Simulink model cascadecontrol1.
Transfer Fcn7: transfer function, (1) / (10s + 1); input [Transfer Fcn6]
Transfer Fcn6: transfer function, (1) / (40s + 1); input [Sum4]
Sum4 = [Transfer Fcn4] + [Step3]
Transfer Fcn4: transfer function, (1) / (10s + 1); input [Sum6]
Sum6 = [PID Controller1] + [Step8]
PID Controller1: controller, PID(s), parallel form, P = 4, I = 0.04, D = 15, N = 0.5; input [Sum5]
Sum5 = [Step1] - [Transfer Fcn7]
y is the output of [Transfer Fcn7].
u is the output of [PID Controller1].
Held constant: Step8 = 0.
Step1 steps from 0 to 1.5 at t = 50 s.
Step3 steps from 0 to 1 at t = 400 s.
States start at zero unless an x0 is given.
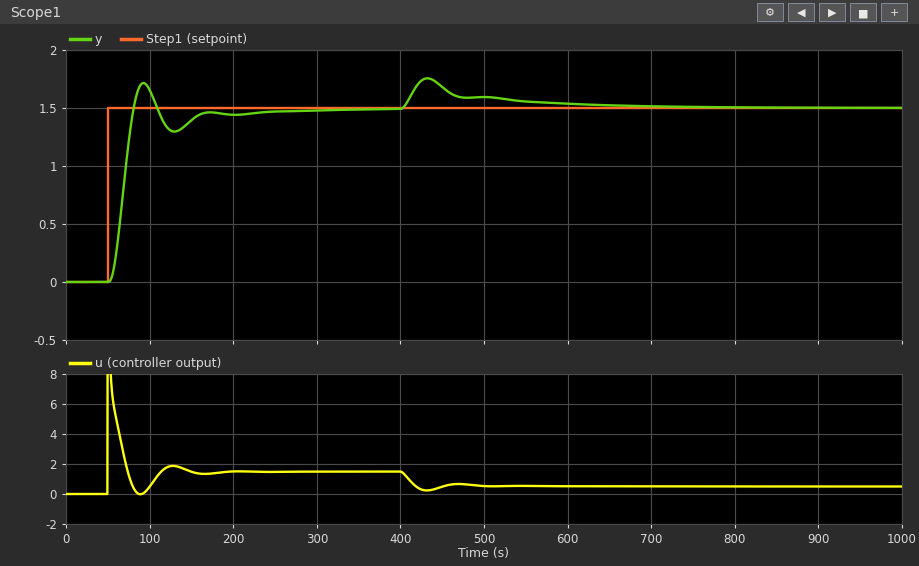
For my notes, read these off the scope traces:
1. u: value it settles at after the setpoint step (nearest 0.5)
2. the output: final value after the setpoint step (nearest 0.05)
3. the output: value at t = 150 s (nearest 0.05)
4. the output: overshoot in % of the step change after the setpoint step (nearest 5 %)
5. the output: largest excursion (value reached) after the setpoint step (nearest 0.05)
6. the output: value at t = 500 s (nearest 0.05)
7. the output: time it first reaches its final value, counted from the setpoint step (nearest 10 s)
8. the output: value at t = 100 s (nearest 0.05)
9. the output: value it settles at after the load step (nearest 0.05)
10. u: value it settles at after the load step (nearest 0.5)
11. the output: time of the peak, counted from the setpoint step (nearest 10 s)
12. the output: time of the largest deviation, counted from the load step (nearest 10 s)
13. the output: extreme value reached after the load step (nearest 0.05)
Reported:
1.5
1.50
1.40
15 %
1.70
1.60
30 s
1.65
1.50
0.5
40 s
30 s
1.75
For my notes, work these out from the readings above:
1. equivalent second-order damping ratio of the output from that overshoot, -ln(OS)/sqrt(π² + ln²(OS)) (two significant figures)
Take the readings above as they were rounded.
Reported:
0.52
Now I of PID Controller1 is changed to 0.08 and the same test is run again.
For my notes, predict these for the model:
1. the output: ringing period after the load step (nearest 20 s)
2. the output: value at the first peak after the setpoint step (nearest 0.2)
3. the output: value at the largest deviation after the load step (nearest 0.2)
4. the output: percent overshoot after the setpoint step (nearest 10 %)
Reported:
80 s
2.0
1.8
30 %
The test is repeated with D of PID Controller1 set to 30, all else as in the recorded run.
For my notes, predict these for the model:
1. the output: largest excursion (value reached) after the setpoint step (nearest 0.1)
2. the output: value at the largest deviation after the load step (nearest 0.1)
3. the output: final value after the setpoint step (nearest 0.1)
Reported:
1.6
1.7
1.5
